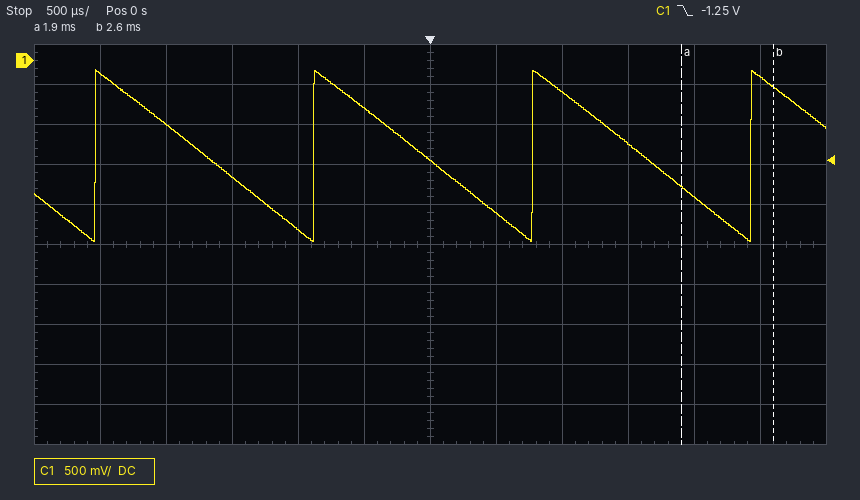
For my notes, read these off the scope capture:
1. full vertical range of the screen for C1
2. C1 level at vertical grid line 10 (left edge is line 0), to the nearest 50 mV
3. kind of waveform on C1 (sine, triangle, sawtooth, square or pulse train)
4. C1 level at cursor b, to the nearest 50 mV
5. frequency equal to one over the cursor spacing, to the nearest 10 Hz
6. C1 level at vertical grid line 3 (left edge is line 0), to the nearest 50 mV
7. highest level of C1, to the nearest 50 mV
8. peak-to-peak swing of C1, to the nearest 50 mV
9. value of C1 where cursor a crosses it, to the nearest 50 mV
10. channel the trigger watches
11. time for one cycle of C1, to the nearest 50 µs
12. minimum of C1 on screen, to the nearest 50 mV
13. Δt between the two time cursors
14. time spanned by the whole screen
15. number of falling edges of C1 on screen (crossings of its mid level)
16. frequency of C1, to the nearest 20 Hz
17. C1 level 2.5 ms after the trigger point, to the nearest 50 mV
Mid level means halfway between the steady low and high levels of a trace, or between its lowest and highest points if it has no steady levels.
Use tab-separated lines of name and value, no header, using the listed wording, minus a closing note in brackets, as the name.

full vertical range of the screen for C1	5 V
C1 level at vertical grid line 10 (left edge is line 0), to the nearest 50 mV	-1.70 V
kind of waveform on C1	sawtooth
C1 level at cursor b, to the nearest 50 mV	-350 mV
frequency equal to one over the cursor spacing, to the nearest 10 Hz	1.43 kHz
C1 level at vertical grid line 3 (left edge is line 0), to the nearest 50 mV	-1.45 V
highest level of C1, to the nearest 50 mV	-100 mV
peak-to-peak swing of C1, to the nearest 50 mV	2.15 V
value of C1 where cursor a crosses it, to the nearest 50 mV	-1.60 V
channel the trigger watches	C1
time for one cycle of C1, to the nearest 50 µs	1.65 ms
minimum of C1 on screen, to the nearest 50 mV	-2.25 V
Δt between the two time cursors	700 µs
time spanned by the whole screen	6 ms
number of falling edges of C1 on screen	3
frequency of C1, to the nearest 20 Hz	600 Hz
C1 level 2.5 ms after the trigger point, to the nearest 50 mV	-200 mV
